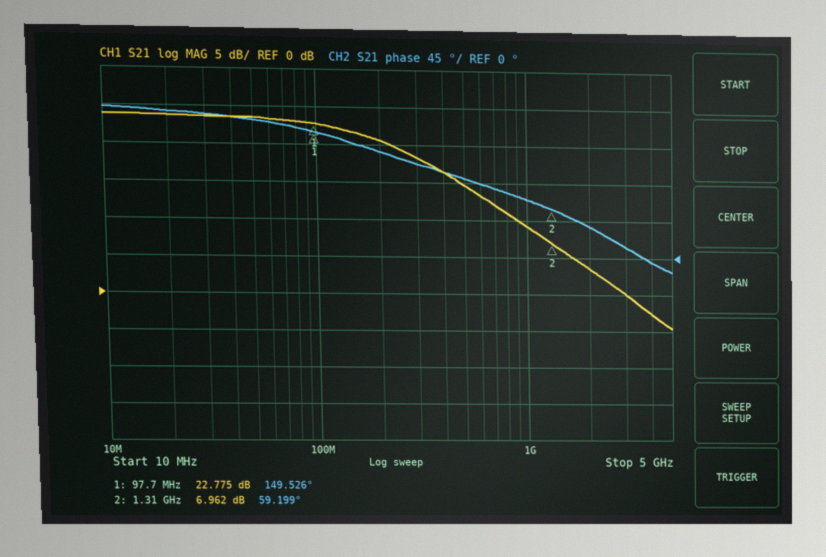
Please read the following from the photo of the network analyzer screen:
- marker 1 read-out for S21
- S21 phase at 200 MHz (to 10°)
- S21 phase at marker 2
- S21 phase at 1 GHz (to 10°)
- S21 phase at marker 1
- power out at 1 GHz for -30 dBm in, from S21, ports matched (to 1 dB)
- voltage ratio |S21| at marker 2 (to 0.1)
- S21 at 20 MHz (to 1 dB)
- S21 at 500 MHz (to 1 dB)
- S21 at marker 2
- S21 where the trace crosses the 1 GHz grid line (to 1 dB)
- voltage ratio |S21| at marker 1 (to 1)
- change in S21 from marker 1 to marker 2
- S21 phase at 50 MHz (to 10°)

22.775 dB
130°
59.199°
70°
149.526°
-21 dBm
2.2
24 dB
15 dB
6.962 dB
9 dB
14
-15.813 dB
160°
